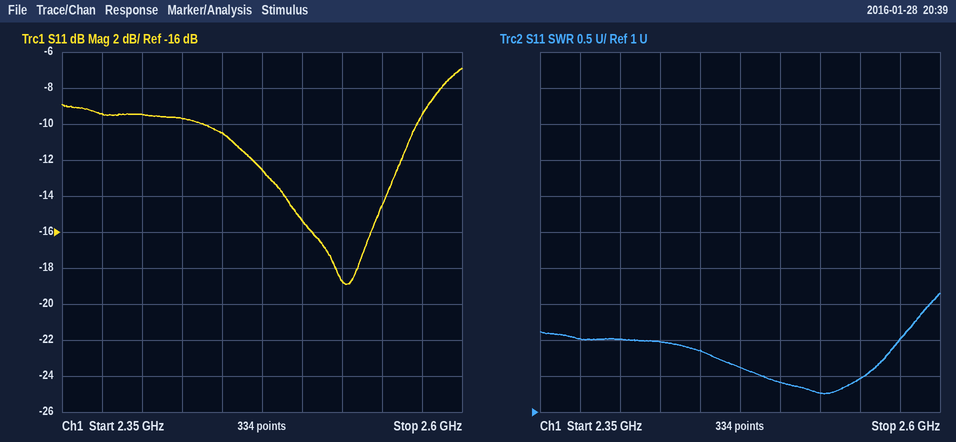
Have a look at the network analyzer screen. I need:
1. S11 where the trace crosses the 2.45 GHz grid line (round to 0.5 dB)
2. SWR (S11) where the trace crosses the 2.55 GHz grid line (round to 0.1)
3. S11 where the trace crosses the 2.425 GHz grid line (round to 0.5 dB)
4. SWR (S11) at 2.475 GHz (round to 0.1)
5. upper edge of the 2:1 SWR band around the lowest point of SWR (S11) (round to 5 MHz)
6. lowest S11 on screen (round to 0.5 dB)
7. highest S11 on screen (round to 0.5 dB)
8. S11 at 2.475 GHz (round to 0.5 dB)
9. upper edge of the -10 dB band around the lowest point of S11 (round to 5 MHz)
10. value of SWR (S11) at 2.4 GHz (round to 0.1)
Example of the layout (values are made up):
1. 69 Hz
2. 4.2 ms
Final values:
1. -10.5 dB
2. 1.5
3. -9.5 dB
4. 1.6
5. 2.575 GHz
6. -19.0 dB
7. -7.0 dB
8. -12.5 dB
9. 2.570 GHz
10. 2.0
